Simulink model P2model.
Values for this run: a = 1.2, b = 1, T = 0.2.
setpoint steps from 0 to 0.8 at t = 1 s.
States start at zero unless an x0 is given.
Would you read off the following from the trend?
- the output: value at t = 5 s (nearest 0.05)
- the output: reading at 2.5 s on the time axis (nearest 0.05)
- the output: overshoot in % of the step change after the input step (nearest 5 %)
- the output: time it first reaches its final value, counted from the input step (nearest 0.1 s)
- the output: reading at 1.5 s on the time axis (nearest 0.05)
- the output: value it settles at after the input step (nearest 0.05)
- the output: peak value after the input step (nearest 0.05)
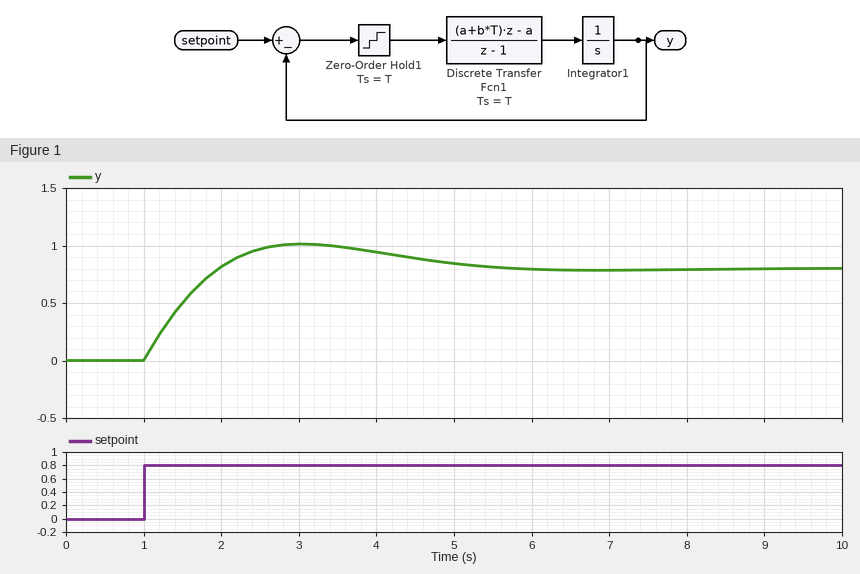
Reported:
0.85
0.95
25 %
1.0 s
0.50
0.80
1.00
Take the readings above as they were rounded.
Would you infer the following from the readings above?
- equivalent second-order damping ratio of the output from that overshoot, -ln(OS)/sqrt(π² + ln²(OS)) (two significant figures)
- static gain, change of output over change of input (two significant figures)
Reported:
0.40
1.0
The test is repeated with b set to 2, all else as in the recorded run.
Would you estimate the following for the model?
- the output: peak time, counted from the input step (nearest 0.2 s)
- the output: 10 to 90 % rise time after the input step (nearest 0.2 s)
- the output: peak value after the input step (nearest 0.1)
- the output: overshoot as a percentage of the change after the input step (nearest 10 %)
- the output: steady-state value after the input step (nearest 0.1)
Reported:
1.6 s
0.6 s
1.1
40 %
0.8
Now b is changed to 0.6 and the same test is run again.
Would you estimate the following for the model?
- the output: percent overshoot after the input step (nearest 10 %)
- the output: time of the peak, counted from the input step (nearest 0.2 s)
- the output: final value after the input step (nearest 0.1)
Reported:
20 %
2.4 s
0.8
